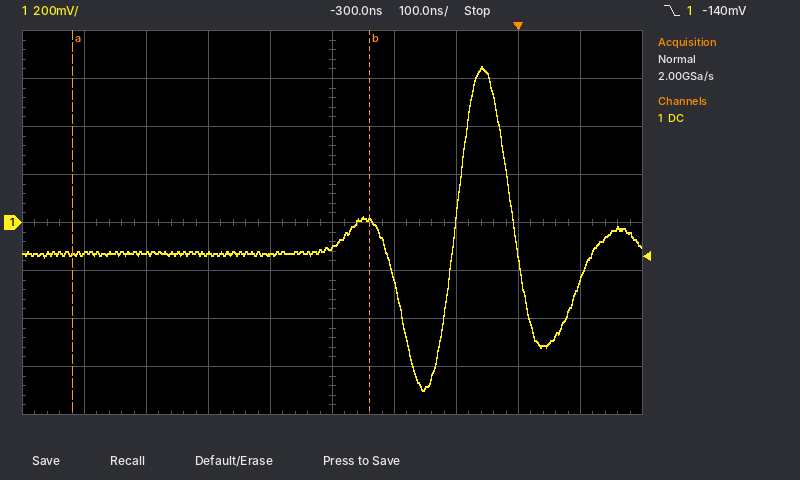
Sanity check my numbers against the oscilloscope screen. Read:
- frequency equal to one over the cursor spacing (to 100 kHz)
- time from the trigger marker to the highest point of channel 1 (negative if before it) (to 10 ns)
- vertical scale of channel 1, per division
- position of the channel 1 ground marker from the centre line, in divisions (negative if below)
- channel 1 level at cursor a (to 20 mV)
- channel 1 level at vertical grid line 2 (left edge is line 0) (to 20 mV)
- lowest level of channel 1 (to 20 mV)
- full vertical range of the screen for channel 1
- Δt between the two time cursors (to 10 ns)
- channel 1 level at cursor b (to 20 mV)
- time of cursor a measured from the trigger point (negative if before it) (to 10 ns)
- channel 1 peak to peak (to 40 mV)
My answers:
2.1 MHz
-60 ns
200 mV
0.0 div
-140 mV
-120 mV
-700 mV
1.6 V
480 ns
0 mV
-720 ns
1.36 V
